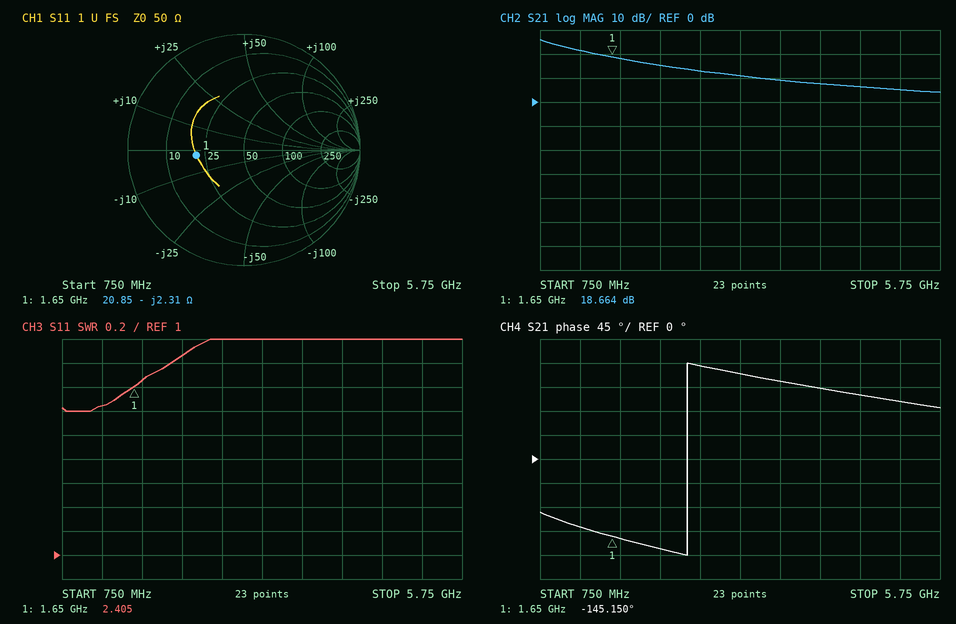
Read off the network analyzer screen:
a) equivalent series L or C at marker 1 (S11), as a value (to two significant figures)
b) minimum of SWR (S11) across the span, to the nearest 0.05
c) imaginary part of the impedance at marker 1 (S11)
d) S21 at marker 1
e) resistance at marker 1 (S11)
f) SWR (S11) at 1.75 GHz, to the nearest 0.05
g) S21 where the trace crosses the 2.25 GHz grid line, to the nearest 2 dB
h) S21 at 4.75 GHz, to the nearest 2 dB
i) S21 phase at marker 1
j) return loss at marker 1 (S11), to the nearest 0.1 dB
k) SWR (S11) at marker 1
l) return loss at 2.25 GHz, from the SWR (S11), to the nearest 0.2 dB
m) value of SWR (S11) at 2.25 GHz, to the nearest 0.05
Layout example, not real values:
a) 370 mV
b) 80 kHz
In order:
a) 42 pF
b) 2.20
c) -2.31 Ω
d) 18.664 dB
e) 20.85 Ω
f) 2.45
g) 16 dB
h) 6 dB
i) -145.150°
j) 7.7 dB
k) 2.405
l) 6.8 dB
m) 2.65
